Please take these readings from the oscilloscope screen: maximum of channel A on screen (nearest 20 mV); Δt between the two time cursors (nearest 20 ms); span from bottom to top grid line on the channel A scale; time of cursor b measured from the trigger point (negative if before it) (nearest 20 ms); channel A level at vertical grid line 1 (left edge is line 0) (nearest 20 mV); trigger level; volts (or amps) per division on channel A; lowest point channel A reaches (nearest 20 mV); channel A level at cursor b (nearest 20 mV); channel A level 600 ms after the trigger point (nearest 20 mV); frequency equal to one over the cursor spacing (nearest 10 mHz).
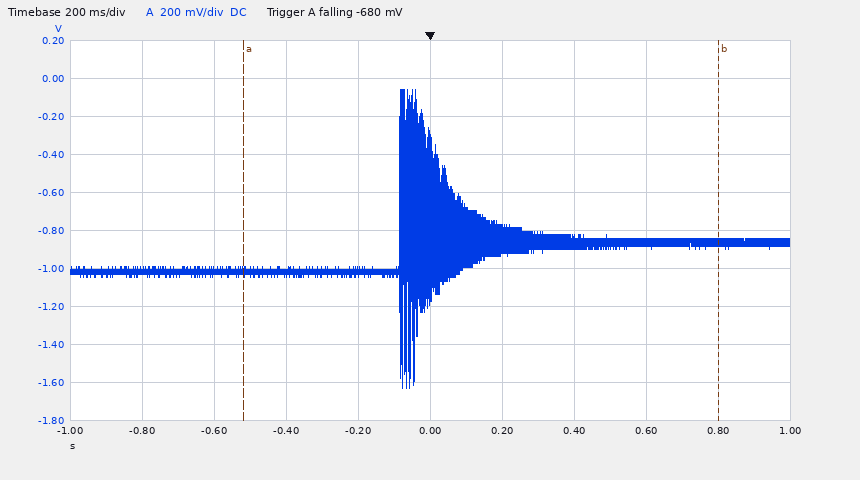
-60 mV
1.32 s
2 V
+800 ms
-1.00 V
-680 mV
200 mV
-1.62 V
-860 mV
-860 mV
760 mHz
